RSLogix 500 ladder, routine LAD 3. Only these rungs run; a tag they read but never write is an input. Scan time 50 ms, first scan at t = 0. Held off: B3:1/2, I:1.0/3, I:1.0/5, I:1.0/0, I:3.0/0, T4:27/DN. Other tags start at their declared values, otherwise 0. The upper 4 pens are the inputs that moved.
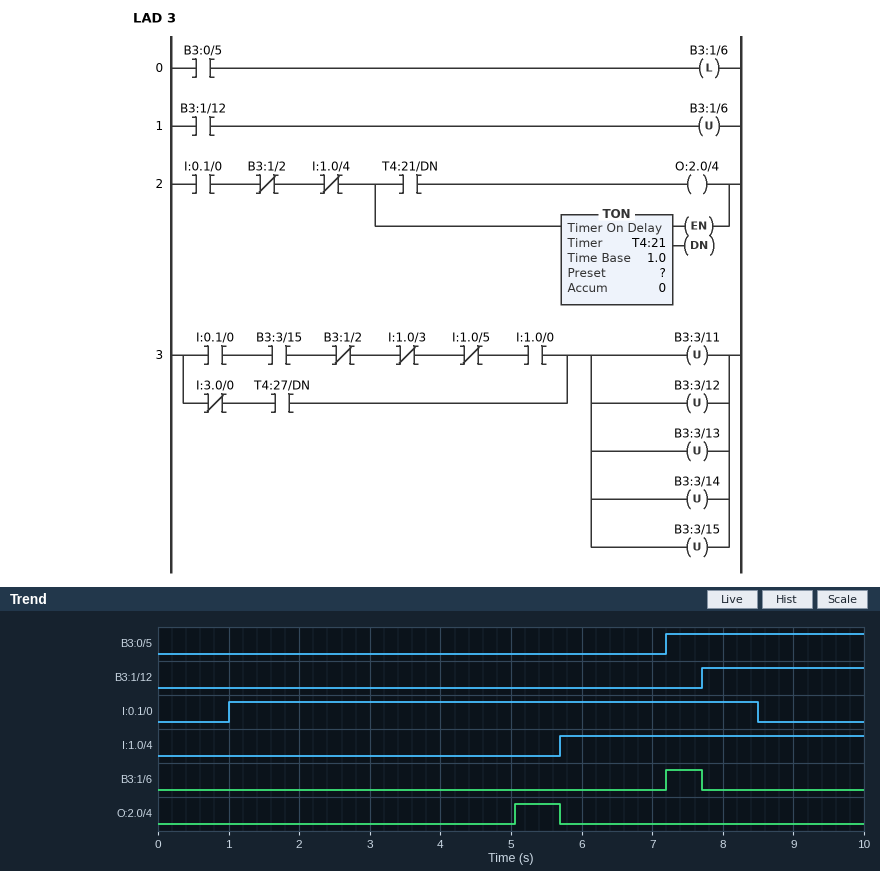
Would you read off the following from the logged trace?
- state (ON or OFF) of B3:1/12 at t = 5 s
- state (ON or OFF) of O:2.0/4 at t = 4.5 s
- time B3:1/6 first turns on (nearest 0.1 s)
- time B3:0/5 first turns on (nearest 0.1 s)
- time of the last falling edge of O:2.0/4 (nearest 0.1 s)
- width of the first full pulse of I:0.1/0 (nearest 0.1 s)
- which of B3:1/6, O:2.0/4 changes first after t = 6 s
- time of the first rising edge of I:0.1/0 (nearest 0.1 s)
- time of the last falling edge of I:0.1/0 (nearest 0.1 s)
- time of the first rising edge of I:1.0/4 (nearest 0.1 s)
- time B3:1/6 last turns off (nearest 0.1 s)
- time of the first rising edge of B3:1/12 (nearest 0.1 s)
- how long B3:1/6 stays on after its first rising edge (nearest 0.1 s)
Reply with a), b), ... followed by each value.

a) OFF
b) OFF
c) 7.2 s
d) 7.2 s
e) 5.7 s
f) 7.5 s
g) B3:1/6
h) 1.0 s
i) 8.5 s
j) 5.7 s
k) 7.7 s
l) 7.7 s
m) 0.5 s
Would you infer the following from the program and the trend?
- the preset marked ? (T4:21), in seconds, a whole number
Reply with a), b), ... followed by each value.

a) 4 s
